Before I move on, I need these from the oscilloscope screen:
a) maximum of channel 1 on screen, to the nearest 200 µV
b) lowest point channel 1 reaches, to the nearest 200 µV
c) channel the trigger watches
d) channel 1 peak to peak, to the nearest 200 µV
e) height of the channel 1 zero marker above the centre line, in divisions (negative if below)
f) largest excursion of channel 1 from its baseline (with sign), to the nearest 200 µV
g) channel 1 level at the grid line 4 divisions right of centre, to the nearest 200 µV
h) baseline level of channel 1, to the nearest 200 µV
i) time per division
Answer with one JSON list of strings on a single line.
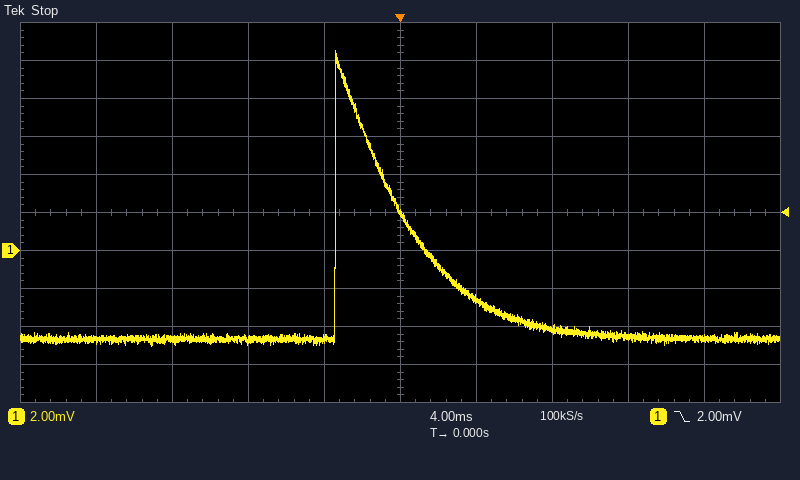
["10.6 mV", "-5.0 mV", "channel 1", "15.6 mV", "-1.0 div", "+15.2 mV", "-4.6 mV", "-4.6 mV", "4 ms"]
